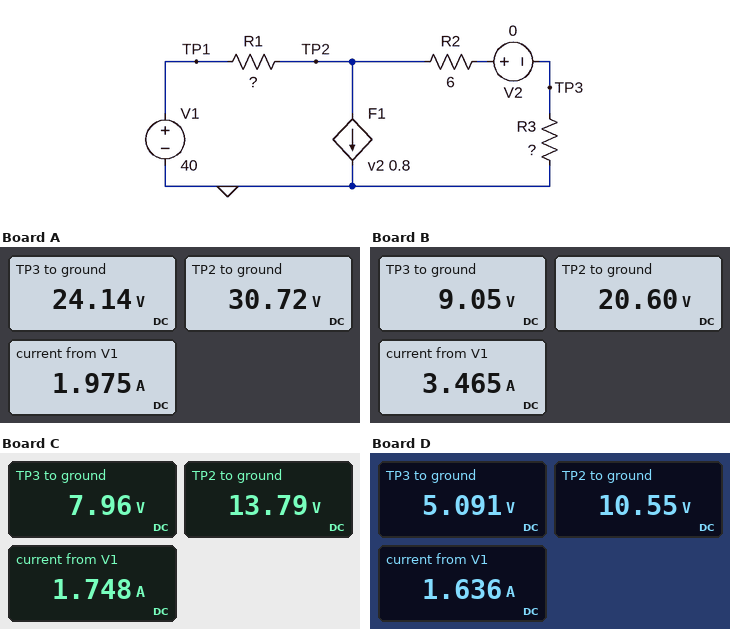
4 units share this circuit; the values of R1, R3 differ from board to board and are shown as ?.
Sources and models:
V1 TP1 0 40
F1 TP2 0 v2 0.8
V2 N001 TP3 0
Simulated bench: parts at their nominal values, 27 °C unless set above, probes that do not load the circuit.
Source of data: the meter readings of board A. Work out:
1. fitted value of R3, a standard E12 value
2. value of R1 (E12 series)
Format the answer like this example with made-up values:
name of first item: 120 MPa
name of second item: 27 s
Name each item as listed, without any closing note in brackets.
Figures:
fitted value of R3, a standard E12 value: 22 Ω
value of R1: 4.7 Ω
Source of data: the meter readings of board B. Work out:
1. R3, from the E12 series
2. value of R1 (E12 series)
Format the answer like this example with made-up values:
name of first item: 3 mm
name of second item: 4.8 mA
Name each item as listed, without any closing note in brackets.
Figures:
R3, from the E12 series: 4.7 Ω
value of R1: 5.6 Ω
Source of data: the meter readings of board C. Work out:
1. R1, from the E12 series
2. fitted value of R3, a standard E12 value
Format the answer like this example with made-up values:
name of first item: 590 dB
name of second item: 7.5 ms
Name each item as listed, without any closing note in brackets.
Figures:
R1, from the E12 series: 15 Ω
fitted value of R3, a standard E12 value: 8.2 Ω
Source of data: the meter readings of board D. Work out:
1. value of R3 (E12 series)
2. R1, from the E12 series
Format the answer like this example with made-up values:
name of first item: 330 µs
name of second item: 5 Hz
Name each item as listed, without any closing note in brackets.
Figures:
value of R3: 5.6 Ω
R1, from the E12 series: 18 Ω
